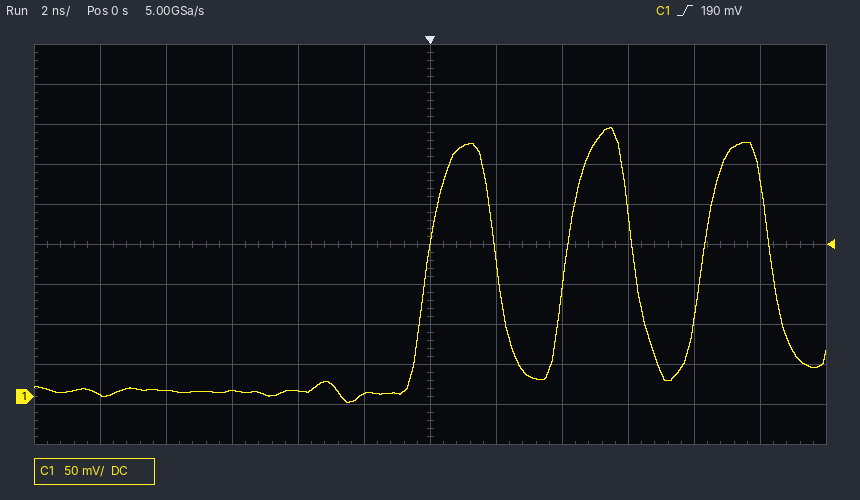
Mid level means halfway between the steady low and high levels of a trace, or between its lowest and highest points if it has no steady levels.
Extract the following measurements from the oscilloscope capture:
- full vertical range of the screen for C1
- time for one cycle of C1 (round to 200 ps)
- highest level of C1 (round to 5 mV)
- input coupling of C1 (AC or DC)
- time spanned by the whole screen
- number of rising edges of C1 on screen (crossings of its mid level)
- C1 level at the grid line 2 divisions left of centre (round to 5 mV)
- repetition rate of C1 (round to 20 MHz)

500 mV
4.2 ns
335 mV
DC
24 ns
3
5 mV
240 MHz
